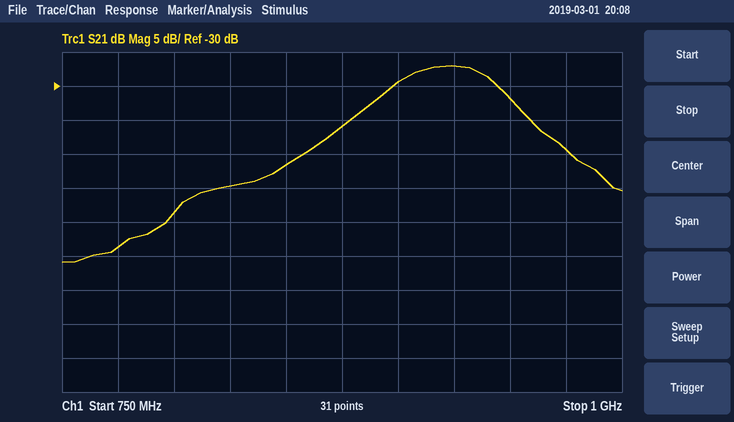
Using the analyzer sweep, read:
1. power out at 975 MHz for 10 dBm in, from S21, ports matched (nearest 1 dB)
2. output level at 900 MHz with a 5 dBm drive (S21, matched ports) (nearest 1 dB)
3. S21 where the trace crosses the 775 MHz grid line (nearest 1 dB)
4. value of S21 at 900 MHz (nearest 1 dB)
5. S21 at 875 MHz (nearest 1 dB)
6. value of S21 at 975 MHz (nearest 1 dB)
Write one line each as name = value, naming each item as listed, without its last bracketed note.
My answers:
power out at 975 MHz for 10 dBm in, from S21, ports matched = -29 dBm
output level at 900 MHz with a 5 dBm drive (S21, matched ports) = -24 dBm
S21 where the trace crosses the 775 MHz grid line = -54 dB
value of S21 at 900 MHz = -29 dB
S21 at 875 MHz = -36 dB
value of S21 at 975 MHz = -39 dB
